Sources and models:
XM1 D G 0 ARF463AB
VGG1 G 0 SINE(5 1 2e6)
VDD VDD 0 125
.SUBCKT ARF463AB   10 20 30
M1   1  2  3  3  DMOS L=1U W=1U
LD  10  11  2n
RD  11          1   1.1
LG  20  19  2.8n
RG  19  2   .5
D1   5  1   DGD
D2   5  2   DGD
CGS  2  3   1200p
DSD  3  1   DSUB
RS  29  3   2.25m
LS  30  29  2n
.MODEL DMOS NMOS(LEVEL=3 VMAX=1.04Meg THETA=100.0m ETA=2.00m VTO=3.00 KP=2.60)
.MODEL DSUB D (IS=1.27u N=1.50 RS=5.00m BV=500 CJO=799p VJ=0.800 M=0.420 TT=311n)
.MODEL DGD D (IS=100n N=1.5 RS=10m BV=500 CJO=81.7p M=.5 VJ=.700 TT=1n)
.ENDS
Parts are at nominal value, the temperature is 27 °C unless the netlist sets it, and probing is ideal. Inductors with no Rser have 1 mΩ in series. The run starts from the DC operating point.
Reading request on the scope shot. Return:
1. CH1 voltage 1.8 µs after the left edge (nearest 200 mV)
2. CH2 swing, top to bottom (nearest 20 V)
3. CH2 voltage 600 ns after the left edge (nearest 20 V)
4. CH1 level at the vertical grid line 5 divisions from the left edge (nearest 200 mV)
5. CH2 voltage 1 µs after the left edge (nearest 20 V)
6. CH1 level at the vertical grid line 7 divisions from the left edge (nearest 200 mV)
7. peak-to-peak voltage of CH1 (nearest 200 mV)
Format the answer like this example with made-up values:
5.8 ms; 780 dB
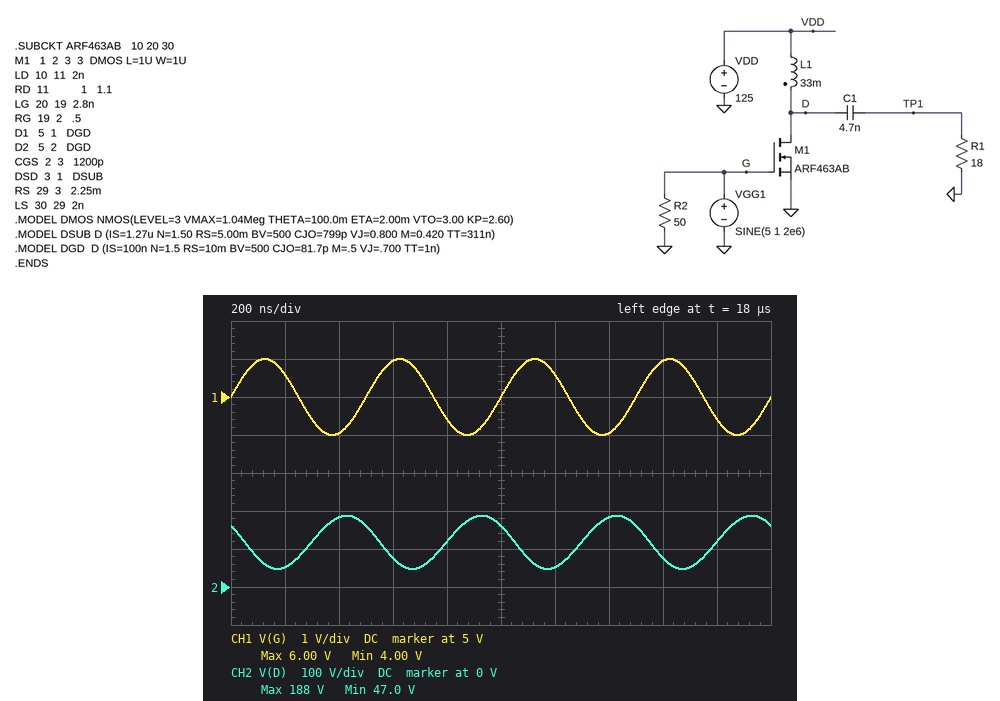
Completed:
4.4 V; 140 V; 80 V; 5.0 V; 160 V; 4.0 V; 2.0 V
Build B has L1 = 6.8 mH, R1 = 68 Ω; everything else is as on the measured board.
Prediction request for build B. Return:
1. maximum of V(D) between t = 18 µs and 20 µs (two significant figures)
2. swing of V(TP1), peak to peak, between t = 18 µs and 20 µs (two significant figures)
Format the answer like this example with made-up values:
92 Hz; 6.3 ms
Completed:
240 V; 230 V
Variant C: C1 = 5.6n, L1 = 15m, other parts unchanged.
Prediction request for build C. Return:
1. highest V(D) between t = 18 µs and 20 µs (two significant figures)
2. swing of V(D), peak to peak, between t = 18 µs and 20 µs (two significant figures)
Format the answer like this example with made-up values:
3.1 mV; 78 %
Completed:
180 V; 130 V
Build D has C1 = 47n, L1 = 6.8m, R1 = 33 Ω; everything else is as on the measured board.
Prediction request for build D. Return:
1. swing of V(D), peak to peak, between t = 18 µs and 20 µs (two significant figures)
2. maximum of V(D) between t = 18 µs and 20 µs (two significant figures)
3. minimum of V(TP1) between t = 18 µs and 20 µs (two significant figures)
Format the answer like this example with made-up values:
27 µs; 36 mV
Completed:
160 V; 200 V; -81 V
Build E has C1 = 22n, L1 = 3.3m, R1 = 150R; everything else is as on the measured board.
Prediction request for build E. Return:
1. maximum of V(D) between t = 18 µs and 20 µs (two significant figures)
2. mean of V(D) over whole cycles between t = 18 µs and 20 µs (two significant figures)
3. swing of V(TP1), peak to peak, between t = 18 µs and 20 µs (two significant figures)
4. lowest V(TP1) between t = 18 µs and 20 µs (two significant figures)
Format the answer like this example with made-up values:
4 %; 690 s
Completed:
280 V; 130 V; 270 V; -120 V
